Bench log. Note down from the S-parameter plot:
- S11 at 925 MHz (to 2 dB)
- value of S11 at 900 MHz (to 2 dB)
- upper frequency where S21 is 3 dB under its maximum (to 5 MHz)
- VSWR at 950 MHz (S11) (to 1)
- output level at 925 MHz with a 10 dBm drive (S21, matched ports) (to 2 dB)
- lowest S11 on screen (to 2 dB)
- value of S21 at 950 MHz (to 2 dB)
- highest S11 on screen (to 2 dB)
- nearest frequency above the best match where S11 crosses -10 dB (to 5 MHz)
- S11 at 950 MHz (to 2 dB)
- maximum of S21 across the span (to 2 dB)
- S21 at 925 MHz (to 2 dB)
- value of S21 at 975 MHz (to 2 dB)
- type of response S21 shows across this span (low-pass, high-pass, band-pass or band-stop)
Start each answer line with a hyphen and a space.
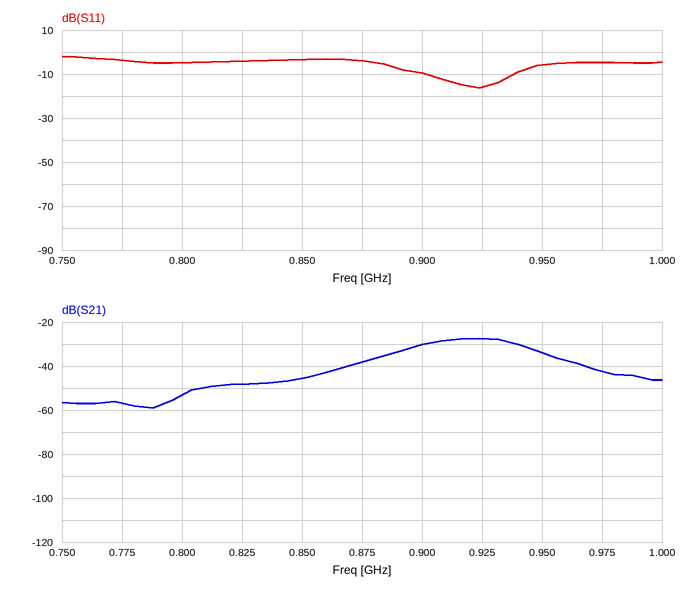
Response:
- -16 dB
- -10 dB
- 940 MHz
- 3
- -18 dBm
- -16 dB
- -34 dB
- -2 dB
- 940 MHz
- -6 dB
- -28 dB
- -28 dB
- -42 dB
- band-pass
